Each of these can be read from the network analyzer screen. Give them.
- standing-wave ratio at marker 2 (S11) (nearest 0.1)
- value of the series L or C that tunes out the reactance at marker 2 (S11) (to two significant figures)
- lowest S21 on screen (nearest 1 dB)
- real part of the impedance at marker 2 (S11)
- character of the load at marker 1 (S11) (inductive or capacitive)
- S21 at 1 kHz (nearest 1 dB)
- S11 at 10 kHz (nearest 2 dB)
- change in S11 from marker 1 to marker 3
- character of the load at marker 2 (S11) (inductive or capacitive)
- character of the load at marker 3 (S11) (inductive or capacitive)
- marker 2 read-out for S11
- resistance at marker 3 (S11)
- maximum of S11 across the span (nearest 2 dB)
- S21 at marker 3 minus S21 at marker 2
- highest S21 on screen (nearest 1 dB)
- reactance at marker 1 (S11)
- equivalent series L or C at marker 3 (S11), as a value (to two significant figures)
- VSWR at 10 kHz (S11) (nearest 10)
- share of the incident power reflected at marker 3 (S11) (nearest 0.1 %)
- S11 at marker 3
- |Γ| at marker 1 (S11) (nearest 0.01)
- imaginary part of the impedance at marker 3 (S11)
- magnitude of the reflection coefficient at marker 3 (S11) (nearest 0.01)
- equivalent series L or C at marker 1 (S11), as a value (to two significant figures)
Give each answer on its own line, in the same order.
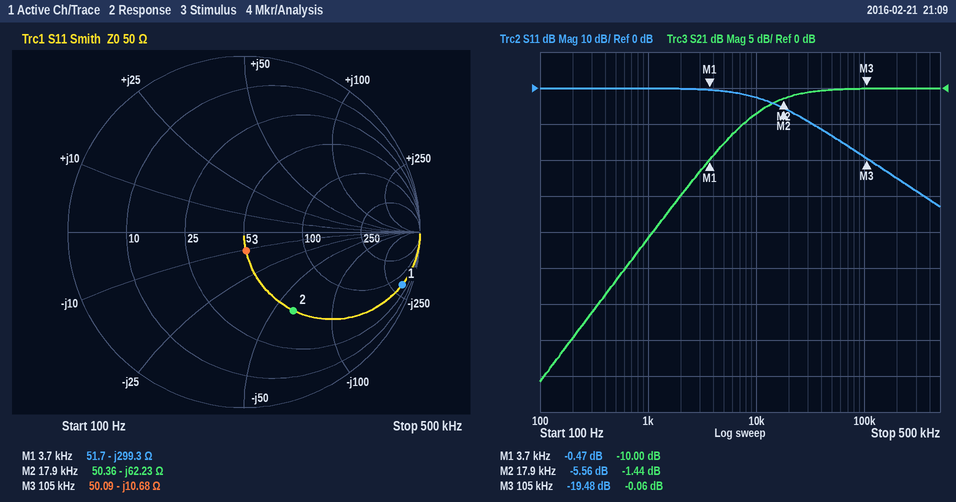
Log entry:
3.2
550 µH
-41 dB
50.36 Ω
capacitive
-21 dB
-2 dB
-19.01 dB
capacitive
capacitive
-5.56 dB
50.09 Ω
0 dB
1.38 dB
0 dB
-299.3 Ω
140 nF
10
1.1 %
-19.48 dB
0.95
-10.68 Ω
0.11
140 nF
